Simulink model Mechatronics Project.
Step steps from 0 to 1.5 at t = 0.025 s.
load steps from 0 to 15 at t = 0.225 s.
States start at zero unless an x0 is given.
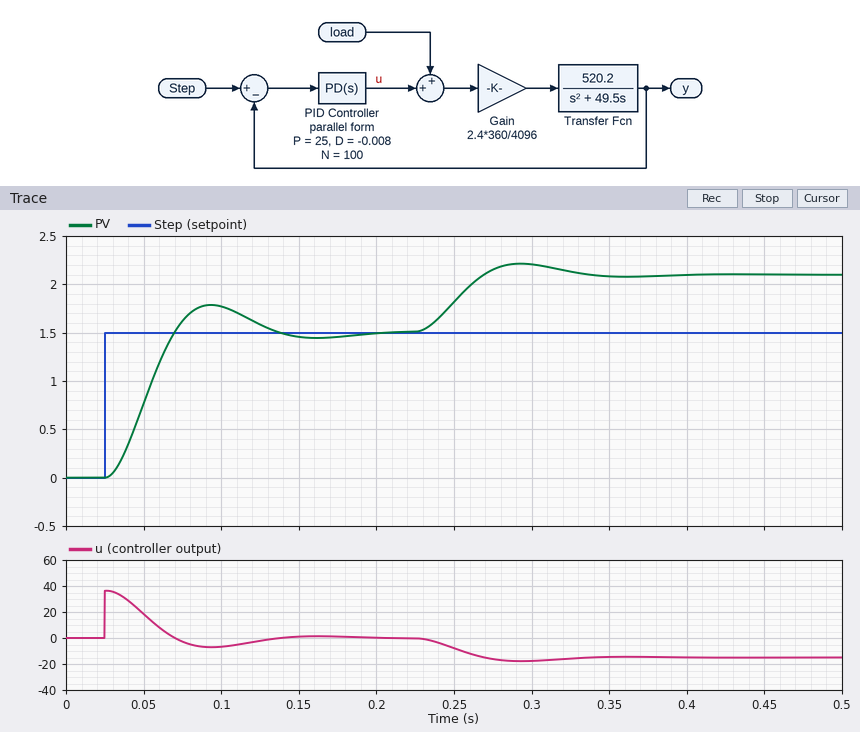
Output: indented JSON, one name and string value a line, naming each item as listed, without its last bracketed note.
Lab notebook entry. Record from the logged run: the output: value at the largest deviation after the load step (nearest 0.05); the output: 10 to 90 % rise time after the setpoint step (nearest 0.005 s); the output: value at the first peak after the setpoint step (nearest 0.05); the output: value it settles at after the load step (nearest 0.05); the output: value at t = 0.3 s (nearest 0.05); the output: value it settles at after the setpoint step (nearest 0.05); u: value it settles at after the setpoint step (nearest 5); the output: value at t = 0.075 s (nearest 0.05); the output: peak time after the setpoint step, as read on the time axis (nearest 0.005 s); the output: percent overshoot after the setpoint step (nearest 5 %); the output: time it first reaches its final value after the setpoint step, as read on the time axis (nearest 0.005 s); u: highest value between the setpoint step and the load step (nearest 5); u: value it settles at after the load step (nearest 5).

{
  "the output: value at the largest deviation after the load step": "2.20",
  "the output: 10 to 90 % rise time after the setpoint step": "0.030 s",
  "the output: value at the first peak after the setpoint step": "1.80",
  "the output: value it settles at after the load step": "2.10",
  "the output: value at t = 0.3 s": "2.20",
  "the output: value it settles at after the setpoint step": "1.50",
  "u: value it settles at after the setpoint step": "0",
  "the output: value at t = 0.075 s": "1.60",
  "the output: peak time after the setpoint step, as read on the time axis": "0.095 s",
  "the output: percent overshoot after the setpoint step": "20 %",
  "the output: time it first reaches its final value after the setpoint step, as read on the time axis": "0.070 s",
  "u: highest value between the setpoint step and the load step": "35",
  "u: value it settles at after the load step": "-15"
}
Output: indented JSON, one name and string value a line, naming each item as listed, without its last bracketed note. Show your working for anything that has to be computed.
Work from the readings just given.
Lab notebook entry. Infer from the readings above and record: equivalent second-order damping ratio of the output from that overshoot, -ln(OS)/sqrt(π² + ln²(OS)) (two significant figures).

{
  "equivalent second-order damping ratio of the output from that overshoot, -ln(OS)/sqrt(π² + ln²(OS))": "ln(0.2) = -1.609; 1.609 / sqrt(9.870 + 2.590) = 0.46"
}
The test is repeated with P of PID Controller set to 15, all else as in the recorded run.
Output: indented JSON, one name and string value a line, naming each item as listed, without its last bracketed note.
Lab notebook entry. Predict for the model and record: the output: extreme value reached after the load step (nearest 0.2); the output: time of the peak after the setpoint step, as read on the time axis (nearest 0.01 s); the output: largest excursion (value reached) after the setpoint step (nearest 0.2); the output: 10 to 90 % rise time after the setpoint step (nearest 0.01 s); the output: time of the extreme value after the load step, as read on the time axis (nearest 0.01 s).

{
  "the output: extreme value reached after the load step": "2.6",
  "the output: time of the peak after the setpoint step, as read on the time axis": "0.12 s",
  "the output: largest excursion (value reached) after the setpoint step": "1.6",
  "the output: 10 to 90 % rise time after the setpoint step": "0.05 s",
  "the output: time of the extreme value after the load step, as read on the time axis": "0.32 s"
}
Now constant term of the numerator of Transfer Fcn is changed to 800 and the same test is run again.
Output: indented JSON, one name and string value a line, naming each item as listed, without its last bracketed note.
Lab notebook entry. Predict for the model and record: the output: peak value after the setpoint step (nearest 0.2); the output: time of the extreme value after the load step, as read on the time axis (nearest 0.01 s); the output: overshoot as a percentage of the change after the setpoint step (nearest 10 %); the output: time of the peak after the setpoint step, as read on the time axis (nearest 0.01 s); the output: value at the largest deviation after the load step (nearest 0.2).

{
  "the output: peak value after the setpoint step": "2.0",
  "the output: time of the extreme value after the load step, as read on the time axis": "0.28 s",
  "the output: overshoot as a percentage of the change after the setpoint step": "30 %",
  "the output: time of the peak after the setpoint step, as read on the time axis": "0.08 s",
  "the output: value at the largest deviation after the load step": "2.2"
}
